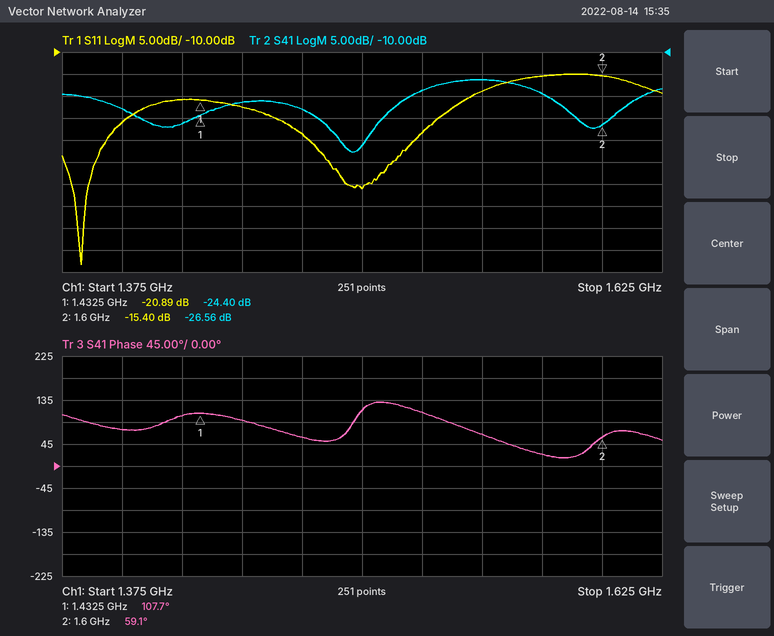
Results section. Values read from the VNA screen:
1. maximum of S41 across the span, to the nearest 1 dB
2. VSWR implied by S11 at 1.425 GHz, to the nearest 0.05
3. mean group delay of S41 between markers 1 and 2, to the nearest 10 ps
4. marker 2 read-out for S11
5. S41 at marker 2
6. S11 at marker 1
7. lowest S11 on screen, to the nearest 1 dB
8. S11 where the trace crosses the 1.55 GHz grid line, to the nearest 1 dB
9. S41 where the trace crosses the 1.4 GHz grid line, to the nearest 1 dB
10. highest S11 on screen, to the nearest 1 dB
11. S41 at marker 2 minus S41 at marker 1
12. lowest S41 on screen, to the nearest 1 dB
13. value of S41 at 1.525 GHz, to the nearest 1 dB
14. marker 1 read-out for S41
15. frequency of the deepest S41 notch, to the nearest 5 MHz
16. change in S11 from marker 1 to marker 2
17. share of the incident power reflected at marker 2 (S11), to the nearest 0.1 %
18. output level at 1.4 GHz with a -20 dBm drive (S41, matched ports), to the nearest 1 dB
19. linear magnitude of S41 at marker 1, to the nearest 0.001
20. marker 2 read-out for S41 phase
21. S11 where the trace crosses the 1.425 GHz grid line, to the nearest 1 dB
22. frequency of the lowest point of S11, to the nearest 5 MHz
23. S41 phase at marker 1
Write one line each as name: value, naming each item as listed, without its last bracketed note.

maximum of S41 across the span, to the nearest 1 dB: -16 dB
VSWR implied by S11 at 1.425 GHz, to the nearest 0.05: 1.20
mean group delay of S41 between markers 1 and 2, to the nearest 10 ps: 810 ps
marker 2 read-out for S11: -15.40 dB
S41 at marker 2: -26.56 dB
S11 at marker 1: -20.89 dB
lowest S11 on screen, to the nearest 1 dB: -58 dB
S11 where the trace crosses the 1.55 GHz grid line, to the nearest 1 dB: -19 dB
S41 where the trace crosses the 1.4 GHz grid line, to the nearest 1 dB: -23 dB
highest S11 on screen, to the nearest 1 dB: -15 dB
S41 at marker 2 minus S41 at marker 1: -2.16 dB
lowest S41 on screen, to the nearest 1 dB: -33 dB
value of S41 at 1.525 GHz, to the nearest 1 dB: -19 dB
marker 1 read-out for S41: -24.40 dB
frequency of the deepest S41 notch, to the nearest 5 MHz: 1.495 GHz
change in S11 from marker 1 to marker 2: 5.49 dB
share of the incident power reflected at marker 2 (S11), to the nearest 0.1 %: 2.9 %
output level at 1.4 GHz with a -20 dBm drive (S41, matched ports), to the nearest 1 dB: -43 dBm
linear magnitude of S41 at marker 1, to the nearest 0.001: 0.060
marker 2 read-out for S41 phase: 59.1°
S11 where the trace crosses the 1.425 GHz grid line, to the nearest 1 dB: -21 dB
frequency of the lowest point of S11, to the nearest 5 MHz: 1.385 GHz
S41 phase at marker 1: 107.7°
